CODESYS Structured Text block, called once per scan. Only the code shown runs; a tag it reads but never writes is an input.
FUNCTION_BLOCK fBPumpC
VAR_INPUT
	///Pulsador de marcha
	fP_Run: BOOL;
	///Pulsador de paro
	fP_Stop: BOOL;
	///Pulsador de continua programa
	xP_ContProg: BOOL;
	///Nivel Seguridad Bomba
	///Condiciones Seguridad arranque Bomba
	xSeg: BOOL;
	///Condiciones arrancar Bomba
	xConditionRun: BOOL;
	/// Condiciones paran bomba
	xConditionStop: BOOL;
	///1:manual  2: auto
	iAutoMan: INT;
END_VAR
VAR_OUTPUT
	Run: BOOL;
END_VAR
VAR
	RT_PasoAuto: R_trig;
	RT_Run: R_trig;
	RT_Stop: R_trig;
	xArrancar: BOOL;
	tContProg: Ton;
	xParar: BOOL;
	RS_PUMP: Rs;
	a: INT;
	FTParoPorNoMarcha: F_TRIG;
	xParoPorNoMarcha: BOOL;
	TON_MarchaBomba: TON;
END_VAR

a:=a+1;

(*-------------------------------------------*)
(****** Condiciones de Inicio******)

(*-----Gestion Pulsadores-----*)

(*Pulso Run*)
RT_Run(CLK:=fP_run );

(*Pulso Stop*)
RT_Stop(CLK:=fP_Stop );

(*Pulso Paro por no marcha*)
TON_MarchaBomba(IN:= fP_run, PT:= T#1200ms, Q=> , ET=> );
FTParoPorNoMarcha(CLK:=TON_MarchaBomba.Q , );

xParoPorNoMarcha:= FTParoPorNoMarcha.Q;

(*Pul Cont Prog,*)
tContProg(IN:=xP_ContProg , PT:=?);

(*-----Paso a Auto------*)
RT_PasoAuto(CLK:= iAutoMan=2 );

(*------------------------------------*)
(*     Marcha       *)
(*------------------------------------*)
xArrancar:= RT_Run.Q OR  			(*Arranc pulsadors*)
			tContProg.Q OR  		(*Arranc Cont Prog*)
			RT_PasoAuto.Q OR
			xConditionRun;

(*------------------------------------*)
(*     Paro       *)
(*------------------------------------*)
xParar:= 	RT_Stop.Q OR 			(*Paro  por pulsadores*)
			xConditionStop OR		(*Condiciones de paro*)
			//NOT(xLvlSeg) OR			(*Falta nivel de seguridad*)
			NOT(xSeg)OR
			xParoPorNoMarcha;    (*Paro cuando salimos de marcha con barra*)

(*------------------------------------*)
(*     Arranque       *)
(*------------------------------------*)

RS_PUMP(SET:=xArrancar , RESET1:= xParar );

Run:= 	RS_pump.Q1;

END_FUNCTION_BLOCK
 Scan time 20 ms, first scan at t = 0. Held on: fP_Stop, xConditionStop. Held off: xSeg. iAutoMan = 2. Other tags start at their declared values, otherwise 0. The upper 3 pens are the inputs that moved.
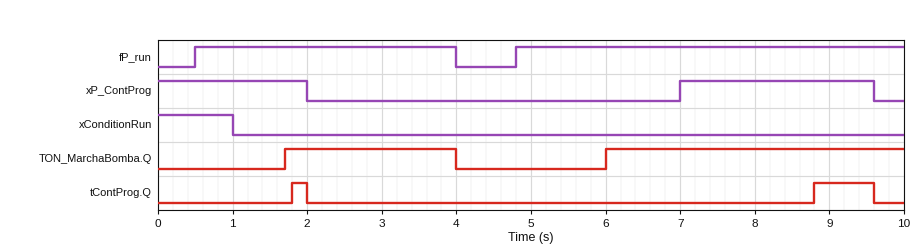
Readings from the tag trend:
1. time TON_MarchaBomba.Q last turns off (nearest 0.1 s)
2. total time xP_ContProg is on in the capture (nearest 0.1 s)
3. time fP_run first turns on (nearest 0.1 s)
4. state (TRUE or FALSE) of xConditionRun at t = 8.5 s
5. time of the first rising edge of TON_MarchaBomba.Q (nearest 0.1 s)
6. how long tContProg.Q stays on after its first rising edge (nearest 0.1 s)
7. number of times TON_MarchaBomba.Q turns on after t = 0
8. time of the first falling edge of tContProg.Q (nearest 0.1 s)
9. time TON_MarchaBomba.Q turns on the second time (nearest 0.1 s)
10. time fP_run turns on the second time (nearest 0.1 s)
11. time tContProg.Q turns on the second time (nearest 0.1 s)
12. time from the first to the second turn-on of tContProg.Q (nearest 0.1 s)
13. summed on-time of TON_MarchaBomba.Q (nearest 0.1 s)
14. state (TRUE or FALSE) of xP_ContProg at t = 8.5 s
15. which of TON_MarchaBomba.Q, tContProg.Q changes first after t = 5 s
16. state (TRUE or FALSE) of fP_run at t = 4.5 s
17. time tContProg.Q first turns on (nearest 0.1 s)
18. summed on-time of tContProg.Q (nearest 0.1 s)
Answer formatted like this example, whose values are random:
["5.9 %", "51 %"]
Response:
["4.0 s", "4.6 s", "0.5 s", "FALSE", "1.7 s", "0.2 s", "2", "2.0 s", "6.0 s", "4.8 s", "8.8 s", "7.0 s", "6.3 s", "TRUE", "TON_MarchaBomba.Q", "FALSE", "1.8 s", "1.0 s"]
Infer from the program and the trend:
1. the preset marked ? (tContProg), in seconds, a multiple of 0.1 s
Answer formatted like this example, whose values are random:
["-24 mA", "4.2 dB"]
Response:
["1.8 s"]
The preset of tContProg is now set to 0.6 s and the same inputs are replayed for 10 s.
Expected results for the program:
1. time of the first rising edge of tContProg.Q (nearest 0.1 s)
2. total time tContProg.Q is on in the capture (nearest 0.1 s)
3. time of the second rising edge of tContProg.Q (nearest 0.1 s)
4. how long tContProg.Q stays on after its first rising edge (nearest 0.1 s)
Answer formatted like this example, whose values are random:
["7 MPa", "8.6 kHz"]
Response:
["0.6 s", "3.4 s", "7.6 s", "1.4 s"]
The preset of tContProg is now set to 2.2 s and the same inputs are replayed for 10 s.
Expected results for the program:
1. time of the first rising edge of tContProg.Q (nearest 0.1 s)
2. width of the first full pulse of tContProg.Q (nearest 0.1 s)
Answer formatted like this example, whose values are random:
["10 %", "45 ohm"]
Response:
["9.2 s", "0.4 s"]
